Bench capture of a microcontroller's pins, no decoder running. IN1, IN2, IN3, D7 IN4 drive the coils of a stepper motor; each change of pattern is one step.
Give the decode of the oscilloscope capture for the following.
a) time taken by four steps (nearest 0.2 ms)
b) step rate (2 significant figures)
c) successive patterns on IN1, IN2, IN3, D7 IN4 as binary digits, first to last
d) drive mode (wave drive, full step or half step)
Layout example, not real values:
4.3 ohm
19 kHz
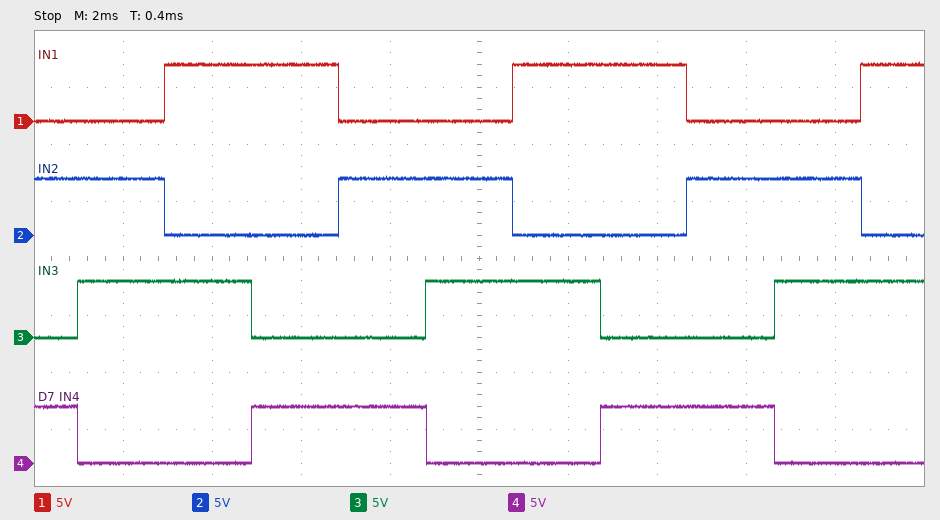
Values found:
7.8 ms
510 steps/s
0101 0110 1010 1001 0101 0110 1010 1001 0101 0110 1010
full step
